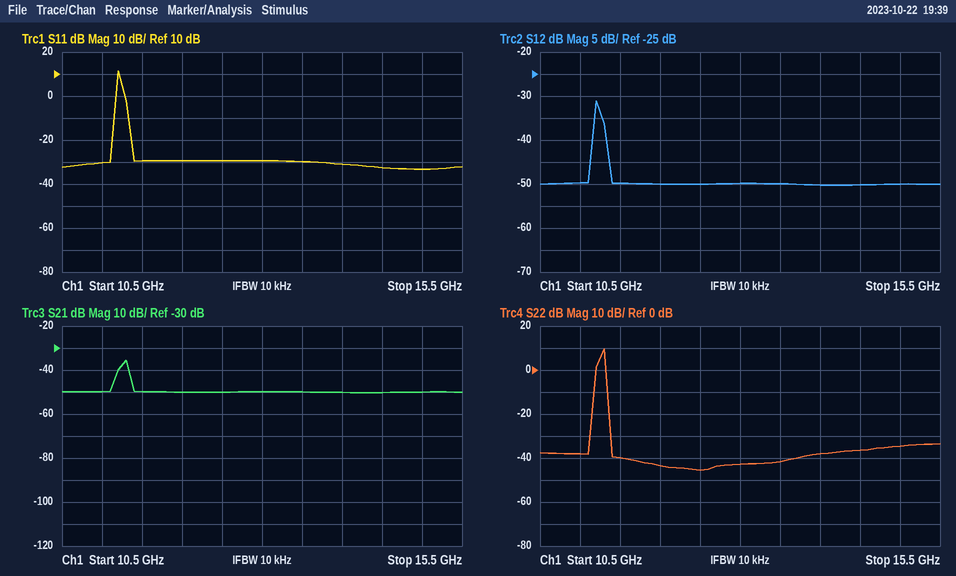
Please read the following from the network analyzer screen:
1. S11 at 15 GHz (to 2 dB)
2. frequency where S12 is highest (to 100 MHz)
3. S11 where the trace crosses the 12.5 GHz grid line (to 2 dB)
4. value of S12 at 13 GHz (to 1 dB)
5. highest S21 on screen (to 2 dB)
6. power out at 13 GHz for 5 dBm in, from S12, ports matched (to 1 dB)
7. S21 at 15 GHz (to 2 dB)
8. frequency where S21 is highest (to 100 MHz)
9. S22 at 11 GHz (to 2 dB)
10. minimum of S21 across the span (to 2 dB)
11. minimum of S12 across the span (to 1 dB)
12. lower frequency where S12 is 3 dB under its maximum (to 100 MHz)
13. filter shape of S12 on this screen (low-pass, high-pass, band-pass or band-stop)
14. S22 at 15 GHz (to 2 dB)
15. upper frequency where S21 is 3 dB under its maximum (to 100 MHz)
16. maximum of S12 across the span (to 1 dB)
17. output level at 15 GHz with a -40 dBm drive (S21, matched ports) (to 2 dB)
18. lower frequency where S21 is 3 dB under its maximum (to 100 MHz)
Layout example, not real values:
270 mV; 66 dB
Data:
-34 dB; 11.2 GHz; -30 dB; -50 dB; -36 dB; -45 dBm; -50 dB; 11.3 GHz; -38 dB; -50 dB; -50 dB; 11.2 GHz; band-pass; -34 dB; 11.3 GHz; -31 dB; -90 dBm; 11.2 GHz
